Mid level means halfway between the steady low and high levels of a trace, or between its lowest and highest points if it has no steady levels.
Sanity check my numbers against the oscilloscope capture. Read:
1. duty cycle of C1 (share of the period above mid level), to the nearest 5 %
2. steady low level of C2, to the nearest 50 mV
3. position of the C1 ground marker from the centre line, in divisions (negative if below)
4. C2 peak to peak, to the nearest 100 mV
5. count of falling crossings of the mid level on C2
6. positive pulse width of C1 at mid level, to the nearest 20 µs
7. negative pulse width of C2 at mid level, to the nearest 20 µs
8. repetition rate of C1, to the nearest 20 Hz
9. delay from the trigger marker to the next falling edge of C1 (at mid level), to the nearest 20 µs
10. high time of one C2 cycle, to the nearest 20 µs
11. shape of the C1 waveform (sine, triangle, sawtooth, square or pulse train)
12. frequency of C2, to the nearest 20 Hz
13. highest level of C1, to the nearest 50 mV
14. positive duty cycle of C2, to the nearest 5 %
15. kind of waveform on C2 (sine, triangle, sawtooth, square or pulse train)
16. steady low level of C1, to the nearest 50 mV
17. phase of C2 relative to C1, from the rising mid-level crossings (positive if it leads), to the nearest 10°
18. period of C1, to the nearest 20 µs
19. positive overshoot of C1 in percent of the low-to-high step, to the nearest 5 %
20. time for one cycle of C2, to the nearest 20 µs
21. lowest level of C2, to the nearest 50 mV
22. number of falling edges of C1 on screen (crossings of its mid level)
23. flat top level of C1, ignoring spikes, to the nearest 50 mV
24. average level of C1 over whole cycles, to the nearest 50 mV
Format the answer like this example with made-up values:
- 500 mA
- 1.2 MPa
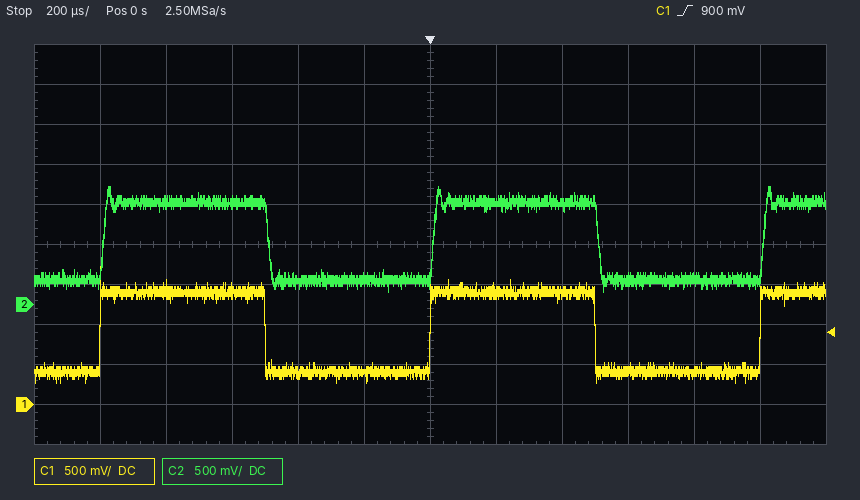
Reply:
- 50 %
- 300 mV
- -4.0 div
- 1.30 V
- 2
- 500 µs
- 500 µs
- 1.00 kHz
- 500 µs
- 500 µs
- square
- 1.00 kHz
- 1.70 V
- 50 %
- square
- 400 mV
- 0°
- 1.00 ms
- 30 %
- 1.00 ms
- 150 mV
- 2
- 1.40 V
- 900 mV
